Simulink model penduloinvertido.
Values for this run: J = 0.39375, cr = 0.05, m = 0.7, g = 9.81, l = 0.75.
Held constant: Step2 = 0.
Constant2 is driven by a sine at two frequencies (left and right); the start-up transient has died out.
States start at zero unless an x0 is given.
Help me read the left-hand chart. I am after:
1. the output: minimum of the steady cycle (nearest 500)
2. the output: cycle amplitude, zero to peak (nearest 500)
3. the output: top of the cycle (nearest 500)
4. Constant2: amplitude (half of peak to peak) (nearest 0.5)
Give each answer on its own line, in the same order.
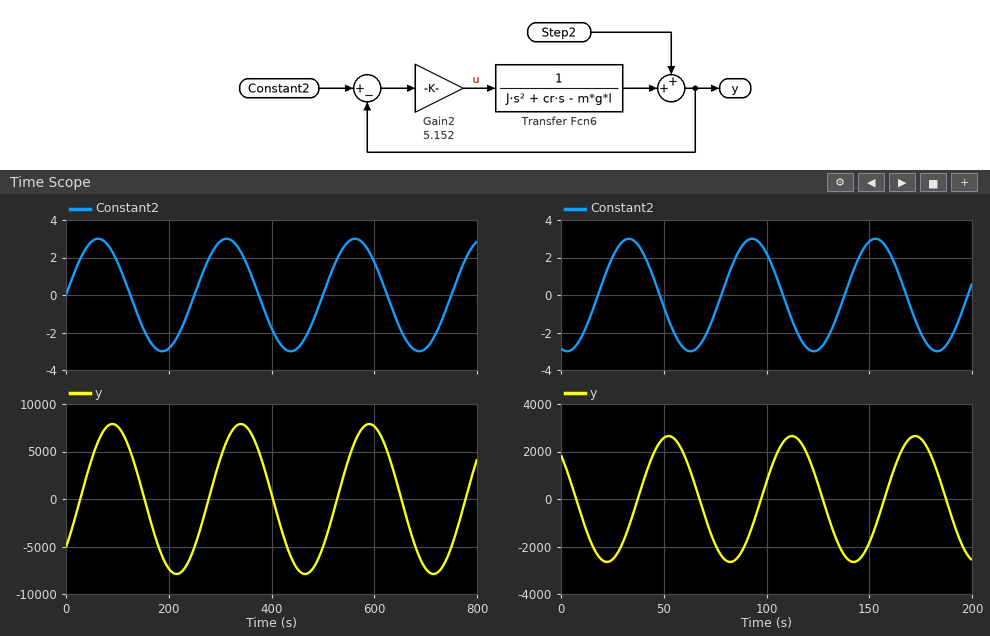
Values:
-8000
8000
8000
3.0
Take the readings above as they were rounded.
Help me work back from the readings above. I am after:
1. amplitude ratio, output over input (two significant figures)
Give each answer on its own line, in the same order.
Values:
2700
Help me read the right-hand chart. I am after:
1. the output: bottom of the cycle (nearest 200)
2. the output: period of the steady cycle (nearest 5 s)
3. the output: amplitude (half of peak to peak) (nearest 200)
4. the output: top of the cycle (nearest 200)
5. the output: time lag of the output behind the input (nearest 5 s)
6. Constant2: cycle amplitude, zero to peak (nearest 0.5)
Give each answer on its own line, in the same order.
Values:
-2600
60 s
2600
2600
20 s
3.0
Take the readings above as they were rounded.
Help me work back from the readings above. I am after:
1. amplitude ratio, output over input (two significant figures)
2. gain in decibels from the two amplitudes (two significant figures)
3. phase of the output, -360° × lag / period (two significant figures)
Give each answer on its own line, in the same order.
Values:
870
59 dB
-120°
